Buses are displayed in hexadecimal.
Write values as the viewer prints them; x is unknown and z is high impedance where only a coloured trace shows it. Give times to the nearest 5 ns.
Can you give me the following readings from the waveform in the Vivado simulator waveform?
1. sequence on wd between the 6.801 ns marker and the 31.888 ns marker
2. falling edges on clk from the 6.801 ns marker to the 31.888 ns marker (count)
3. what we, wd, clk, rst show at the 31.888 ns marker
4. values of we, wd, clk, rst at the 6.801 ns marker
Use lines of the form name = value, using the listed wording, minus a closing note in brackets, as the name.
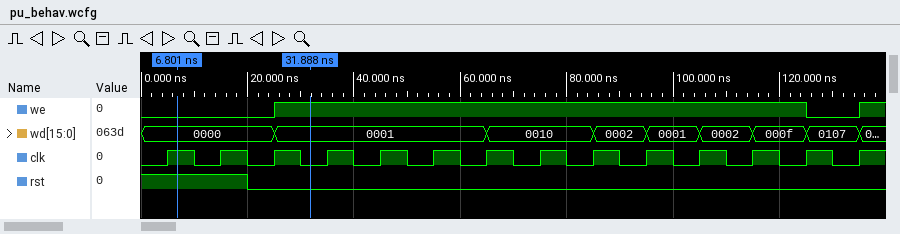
sequence on wd between the 6.801 ns marker and the 31.888 ns marker = 0000, 0001
falling edges on clk from the 6.801 ns marker to the 31.888 ns marker = 3
what we, wd, clk, rst show at the 31.888 ns marker = we=1, wd=0001, clk=0, rst=0
values of we, wd, clk, rst at the 6.801 ns marker = we=0, wd=0000, clk=1, rst=1
